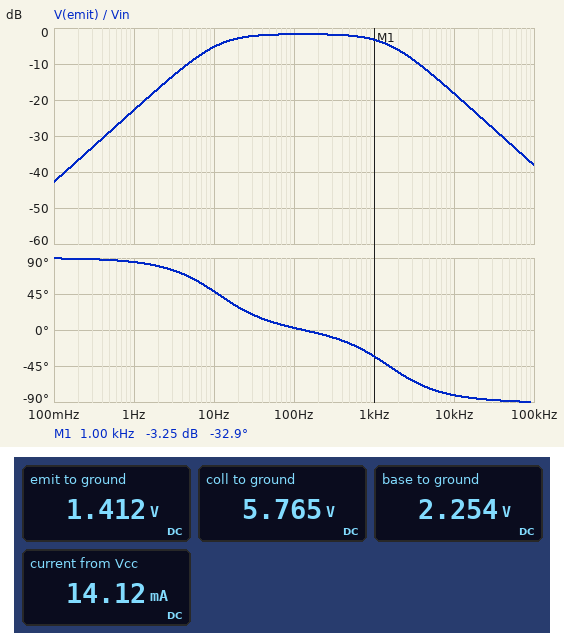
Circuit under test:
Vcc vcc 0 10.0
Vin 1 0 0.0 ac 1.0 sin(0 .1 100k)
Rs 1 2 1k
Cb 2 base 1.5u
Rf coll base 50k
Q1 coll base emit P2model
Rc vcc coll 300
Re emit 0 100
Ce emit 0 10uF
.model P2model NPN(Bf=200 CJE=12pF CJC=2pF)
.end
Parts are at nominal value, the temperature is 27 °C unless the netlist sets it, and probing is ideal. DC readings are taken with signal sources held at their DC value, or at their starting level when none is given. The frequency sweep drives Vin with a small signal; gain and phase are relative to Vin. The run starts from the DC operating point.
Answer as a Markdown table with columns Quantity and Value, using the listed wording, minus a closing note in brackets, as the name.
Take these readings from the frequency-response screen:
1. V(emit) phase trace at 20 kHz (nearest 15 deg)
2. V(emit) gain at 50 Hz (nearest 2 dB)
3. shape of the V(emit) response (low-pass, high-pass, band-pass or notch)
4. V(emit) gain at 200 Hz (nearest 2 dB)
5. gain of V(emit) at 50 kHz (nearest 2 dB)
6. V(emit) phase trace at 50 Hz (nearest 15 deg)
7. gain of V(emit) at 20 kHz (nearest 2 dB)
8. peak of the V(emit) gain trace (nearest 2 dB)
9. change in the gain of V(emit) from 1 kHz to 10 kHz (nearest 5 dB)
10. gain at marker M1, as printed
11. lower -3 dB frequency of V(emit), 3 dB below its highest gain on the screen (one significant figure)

| Quantity | Value |
|---|---|
| V(emit) phase trace at 20 kHz | -90 deg |
| V(emit) gain at 50 Hz | -2 dB |
| shape of the V(emit) response | band-pass |
| V(emit) gain at 200 Hz | -2 dB |
| gain of V(emit) at 50 kHz | -32 dB |
| V(emit) phase trace at 50 Hz | 15 deg |
| gain of V(emit) at 20 kHz | -24 dB |
| peak of the V(emit) gain trace | -2 dB |
| change in the gain of V(emit) from 1 kHz to 10 kHz | -15 dB |
| gain at marker M1, as printed | -3.25 dB |
| lower -3 dB frequency of V(emit), 3 dB below its highest gain on the screen | 10 Hz |
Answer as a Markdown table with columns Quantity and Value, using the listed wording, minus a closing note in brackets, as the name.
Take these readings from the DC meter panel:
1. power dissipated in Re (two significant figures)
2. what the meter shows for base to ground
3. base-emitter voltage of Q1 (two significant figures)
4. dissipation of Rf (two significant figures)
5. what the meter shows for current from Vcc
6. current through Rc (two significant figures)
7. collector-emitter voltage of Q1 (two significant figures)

| Quantity | Value |
|---|---|
| power dissipated in Re | 20 mW |
| what the meter shows for base to ground | 2.254 V |
| base-emitter voltage of Q1 | 840 mV |
| dissipation of Rf | 250 µW |
| what the meter shows for current from Vcc | 14.12 mA |
| current through Rc | 14 mA |
| collector-emitter voltage of Q1 | 4.4 V |
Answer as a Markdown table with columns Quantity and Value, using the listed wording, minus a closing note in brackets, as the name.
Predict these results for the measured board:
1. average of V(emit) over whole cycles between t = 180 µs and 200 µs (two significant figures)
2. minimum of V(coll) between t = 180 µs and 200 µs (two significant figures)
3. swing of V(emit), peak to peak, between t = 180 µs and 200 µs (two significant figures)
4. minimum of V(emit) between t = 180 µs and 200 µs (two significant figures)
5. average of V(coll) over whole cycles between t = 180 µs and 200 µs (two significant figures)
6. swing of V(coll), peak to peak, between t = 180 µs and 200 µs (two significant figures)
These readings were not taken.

| Quantity | Value |
|---|---|
| average of V(emit) over whole cycles between t = 180 µs and 200 µs | 1.4 V |
| minimum of V(coll) between t = 180 µs and 200 µs | 3.4 V |
| swing of V(emit), peak to peak, between t = 180 µs and 200 µs | 2.5 mV |
| minimum of V(emit) between t = 180 µs and 200 µs | 1.4 V |
| average of V(coll) over whole cycles between t = 180 µs and 200 µs | 5.8 V |
| swing of V(coll), peak to peak, between t = 180 µs and 200 µs | 4.6 V |
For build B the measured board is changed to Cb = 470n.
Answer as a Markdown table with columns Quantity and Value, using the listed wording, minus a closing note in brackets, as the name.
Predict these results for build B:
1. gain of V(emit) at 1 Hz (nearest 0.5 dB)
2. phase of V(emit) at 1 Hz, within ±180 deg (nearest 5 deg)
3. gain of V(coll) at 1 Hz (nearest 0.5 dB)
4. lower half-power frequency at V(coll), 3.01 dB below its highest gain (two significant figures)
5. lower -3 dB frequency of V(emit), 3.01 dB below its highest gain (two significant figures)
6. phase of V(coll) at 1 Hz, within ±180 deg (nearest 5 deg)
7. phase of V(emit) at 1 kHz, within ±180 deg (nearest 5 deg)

| Quantity | Value |
|---|---|
| gain of V(emit) at 1 Hz | -33.0 dB |
| phase of V(emit) at 1 Hz, within ±180 deg | 90 deg |
| gain of V(coll) at 1 Hz | -23.5 dB |
| lower half-power frequency at V(coll), 3.01 dB below its highest gain | 1.7 kHz |
| lower -3 dB frequency of V(emit), 3.01 dB below its highest gain | 31 Hz |
| phase of V(coll) at 1 Hz, within ±180 deg | -90 deg |
| phase of V(emit) at 1 kHz, within ±180 deg | -30 deg |
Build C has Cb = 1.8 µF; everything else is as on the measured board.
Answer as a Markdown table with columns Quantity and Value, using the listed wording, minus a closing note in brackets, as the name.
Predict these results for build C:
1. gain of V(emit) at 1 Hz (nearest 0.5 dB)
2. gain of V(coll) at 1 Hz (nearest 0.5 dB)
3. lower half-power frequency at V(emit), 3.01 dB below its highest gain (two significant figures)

| Quantity | Value |
|---|---|
| gain of V(emit) at 1 Hz | -21.0 dB |
| gain of V(coll) at 1 Hz | -12.0 dB |
| lower half-power frequency at V(emit), 3.01 dB below its highest gain | 9.4 Hz |
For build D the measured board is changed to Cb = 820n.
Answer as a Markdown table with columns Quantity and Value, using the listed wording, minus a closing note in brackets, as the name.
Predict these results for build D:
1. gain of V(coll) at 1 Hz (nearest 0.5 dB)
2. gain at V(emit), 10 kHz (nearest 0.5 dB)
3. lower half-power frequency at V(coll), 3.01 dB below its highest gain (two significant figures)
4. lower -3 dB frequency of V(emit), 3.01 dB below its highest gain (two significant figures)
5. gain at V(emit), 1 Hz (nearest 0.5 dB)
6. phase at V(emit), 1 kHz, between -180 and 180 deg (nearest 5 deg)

| Quantity | Value |
|---|---|
| gain of V(coll) at 1 Hz | -18.5 dB |
| gain at V(emit), 10 kHz | -18.0 dB |
| lower half-power frequency at V(coll), 3.01 dB below its highest gain | 1.6 kHz |
| lower -3 dB frequency of V(emit), 3.01 dB below its highest gain | 19 Hz |
| gain at V(emit), 1 Hz | -28.0 dB |
| phase at V(emit), 1 kHz, between -180 and 180 deg | -30 deg |
